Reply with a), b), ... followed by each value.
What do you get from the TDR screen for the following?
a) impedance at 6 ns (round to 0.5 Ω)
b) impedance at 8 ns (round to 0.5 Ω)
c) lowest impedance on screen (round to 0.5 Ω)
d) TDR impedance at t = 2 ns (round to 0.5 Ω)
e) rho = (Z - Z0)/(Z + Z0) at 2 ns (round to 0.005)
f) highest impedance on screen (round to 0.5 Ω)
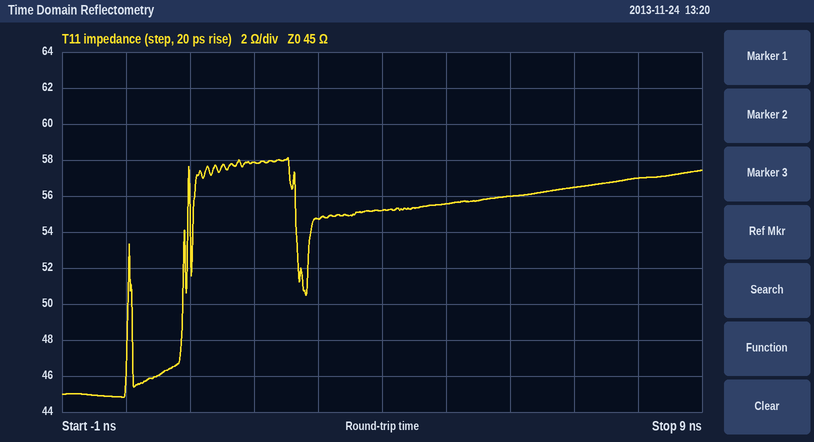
a) 56.0 Ω
b) 57.0 Ω
c) 45.0 Ω
d) 58.0 Ω
e) +0.125
f) 58.0 Ω
